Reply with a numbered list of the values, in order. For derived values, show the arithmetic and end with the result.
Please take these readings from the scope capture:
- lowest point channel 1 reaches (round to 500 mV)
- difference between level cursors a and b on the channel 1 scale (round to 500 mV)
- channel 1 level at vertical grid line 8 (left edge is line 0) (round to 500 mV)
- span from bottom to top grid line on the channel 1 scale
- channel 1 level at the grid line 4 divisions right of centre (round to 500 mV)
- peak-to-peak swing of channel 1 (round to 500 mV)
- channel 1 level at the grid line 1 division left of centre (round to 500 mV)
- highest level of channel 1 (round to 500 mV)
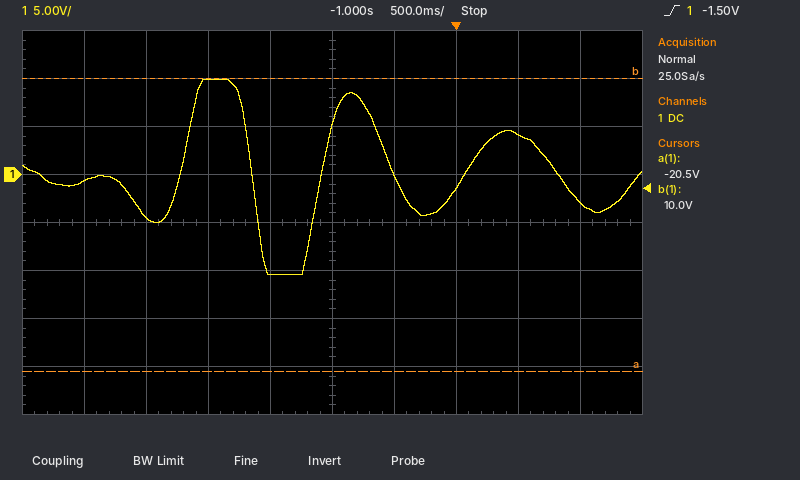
1. -10.5 V
2. 30.5 V
3. 4.0 V
4. 40 V
5. -3.0 V
6. 10.0 V − (-10.5 V) = 20.5 V
7. -10.5 V
8. 10.0 V
